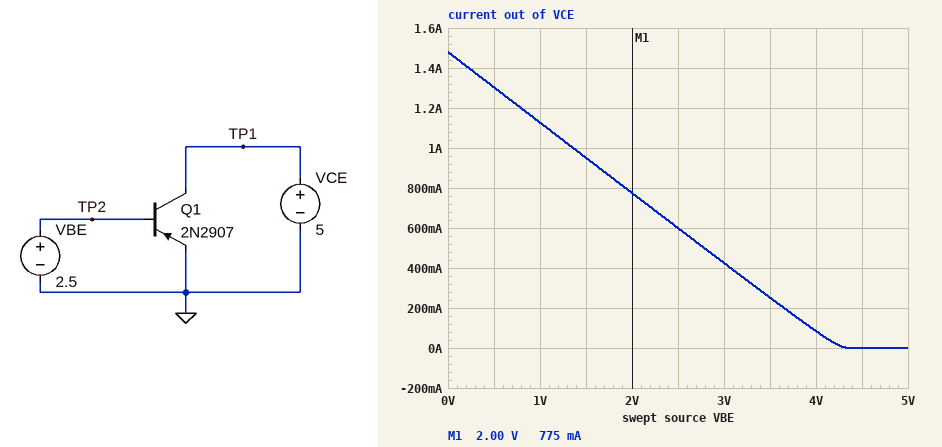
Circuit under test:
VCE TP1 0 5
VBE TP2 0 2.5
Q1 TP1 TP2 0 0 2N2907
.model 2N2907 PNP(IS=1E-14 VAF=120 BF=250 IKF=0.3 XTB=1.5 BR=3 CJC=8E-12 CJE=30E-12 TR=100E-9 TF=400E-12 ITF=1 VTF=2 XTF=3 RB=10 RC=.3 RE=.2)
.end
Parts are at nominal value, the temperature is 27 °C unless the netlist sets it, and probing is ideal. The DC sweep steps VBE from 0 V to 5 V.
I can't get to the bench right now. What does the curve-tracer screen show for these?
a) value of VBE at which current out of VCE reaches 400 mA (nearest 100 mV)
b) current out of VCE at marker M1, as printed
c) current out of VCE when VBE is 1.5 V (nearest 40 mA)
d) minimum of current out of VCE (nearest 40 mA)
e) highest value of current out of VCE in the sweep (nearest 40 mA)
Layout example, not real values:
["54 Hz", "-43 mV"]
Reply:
["3.1 V", "775 mA", "960 mA", "0 A", "1.48 A"]
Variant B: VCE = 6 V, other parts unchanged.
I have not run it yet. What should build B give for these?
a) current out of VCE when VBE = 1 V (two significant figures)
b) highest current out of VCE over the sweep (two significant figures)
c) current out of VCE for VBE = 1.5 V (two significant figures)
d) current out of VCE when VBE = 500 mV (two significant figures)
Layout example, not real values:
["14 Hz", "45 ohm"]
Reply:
["1.5 A", "1.8 A", "1.3 A", "1.7 A"]
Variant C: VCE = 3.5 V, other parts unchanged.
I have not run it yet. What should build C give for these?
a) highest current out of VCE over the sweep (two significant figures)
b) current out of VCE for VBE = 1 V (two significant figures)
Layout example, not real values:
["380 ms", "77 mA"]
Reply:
["950 mA", "600 mA"]
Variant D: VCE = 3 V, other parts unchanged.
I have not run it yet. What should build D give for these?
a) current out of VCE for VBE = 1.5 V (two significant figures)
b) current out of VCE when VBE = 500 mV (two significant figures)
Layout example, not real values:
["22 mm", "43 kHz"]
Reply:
["250 mA", "600 mA"]
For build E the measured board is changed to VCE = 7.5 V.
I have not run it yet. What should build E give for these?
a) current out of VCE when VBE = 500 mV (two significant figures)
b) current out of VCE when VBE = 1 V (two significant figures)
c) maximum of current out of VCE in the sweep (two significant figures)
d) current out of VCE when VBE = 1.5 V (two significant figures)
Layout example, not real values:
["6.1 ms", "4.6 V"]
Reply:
["2.2 A", "2.0 A", "2.4 A", "1.8 A"]
